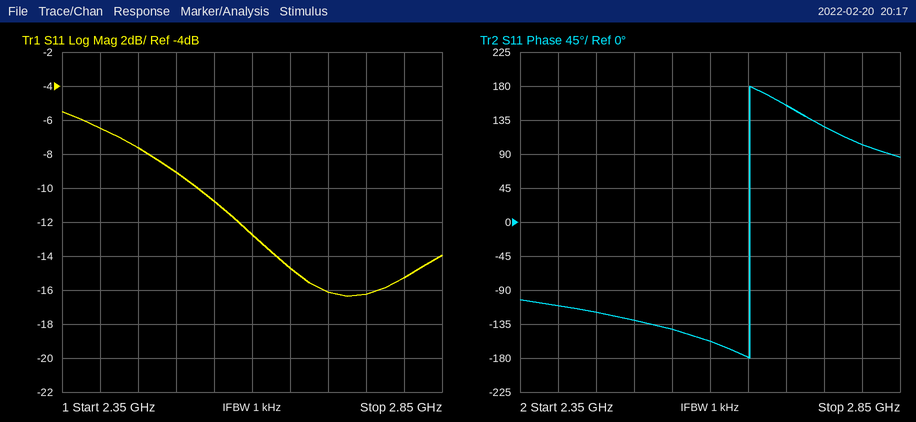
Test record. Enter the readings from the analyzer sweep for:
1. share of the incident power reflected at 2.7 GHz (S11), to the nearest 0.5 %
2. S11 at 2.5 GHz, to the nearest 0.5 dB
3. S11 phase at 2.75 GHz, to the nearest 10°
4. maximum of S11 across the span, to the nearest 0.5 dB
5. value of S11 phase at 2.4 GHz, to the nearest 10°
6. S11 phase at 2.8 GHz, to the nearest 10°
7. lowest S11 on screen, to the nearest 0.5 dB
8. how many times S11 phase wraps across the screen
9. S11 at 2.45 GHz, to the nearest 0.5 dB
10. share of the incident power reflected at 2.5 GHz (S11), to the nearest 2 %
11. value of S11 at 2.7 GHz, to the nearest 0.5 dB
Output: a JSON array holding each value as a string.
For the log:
["2.5 %", "-9.0 dB", "130°", "-5.5 dB", "-110°", "100°", "-16.5 dB", "1", "-7.5 dB", "12 %", "-16.0 dB"]
